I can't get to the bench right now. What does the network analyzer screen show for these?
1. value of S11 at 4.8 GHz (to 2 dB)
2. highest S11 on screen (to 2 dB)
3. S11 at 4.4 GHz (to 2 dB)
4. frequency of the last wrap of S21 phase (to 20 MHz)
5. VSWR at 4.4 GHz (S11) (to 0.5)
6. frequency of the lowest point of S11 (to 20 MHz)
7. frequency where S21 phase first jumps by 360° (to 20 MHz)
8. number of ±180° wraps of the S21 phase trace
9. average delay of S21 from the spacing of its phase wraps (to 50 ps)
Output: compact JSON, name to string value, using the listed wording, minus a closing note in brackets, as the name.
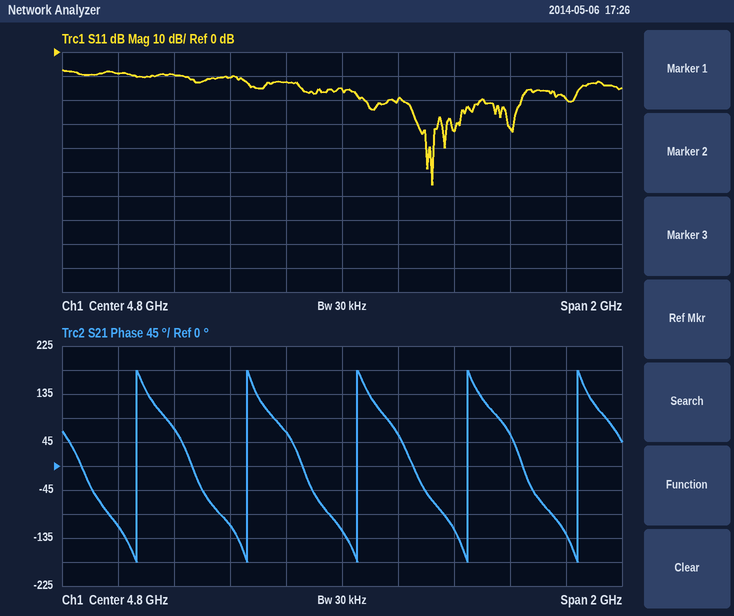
{"value of S11 at 4.8 GHz": "-16 dB", "highest S11 on screen": "-8 dB", "S11 at 4.4 GHz": "-10 dB", "frequency of the last wrap of S21 phase": "5.64 GHz", "VSWR at 4.4 GHz (S11)": "2.0", "frequency of the lowest point of S11": "5.12 GHz", "frequency where S21 phase first jumps by 360°": "4.06 GHz", "number of ±180° wraps of the S21 phase trace": "5", "average delay of S21 from the spacing of its phase wraps": "2.55 ns"}
